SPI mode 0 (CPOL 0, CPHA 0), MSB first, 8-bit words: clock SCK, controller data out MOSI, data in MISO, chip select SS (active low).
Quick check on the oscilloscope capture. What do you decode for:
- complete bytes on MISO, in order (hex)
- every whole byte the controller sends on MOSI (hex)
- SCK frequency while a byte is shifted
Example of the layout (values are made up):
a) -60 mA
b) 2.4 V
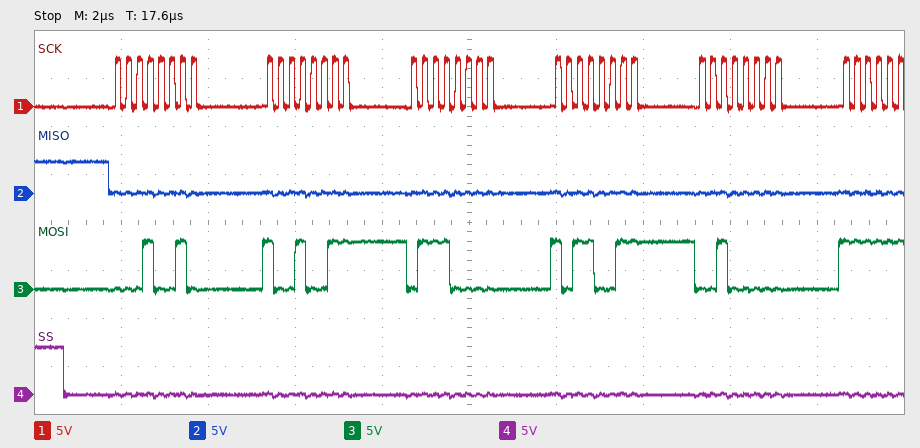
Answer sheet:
a) 00 00 00 00 00
b) 12 93 70 B3 20
c) 4 MHz
